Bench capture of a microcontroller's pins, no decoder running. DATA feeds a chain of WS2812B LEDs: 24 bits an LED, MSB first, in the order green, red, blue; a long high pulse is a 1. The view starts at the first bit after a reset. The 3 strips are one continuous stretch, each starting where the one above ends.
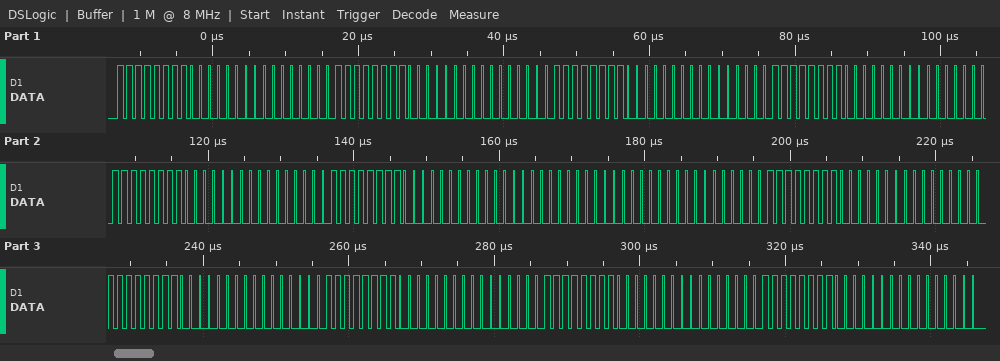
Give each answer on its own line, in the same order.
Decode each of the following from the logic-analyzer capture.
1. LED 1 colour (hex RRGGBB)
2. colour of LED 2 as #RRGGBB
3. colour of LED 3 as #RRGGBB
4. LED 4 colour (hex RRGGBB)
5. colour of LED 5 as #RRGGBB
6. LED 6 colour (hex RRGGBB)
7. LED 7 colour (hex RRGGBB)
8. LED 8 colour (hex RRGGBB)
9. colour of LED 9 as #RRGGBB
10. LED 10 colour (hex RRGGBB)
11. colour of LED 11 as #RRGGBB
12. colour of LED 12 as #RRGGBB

#00FF00
#00FF00
#00FF00
#00FF00
#00FF00
#00FF00
#000000
#00FF00
#00FF00
#00FF00
#00FF00
#00FF00
